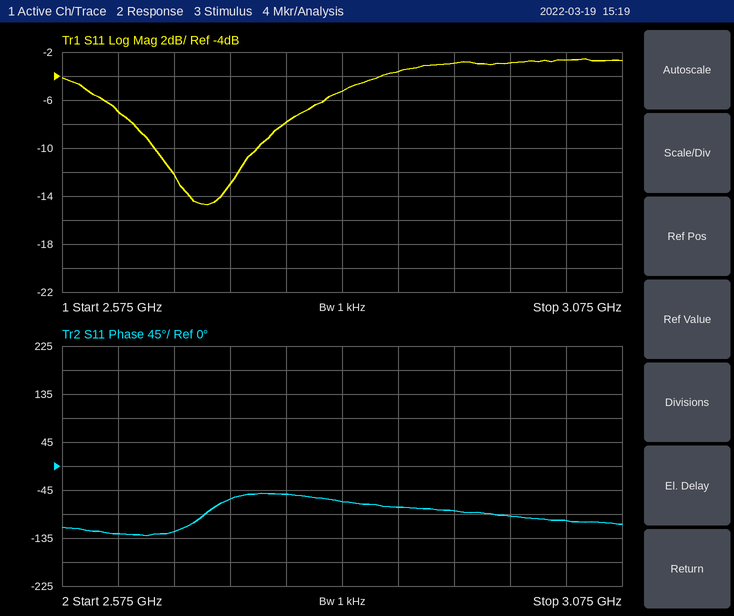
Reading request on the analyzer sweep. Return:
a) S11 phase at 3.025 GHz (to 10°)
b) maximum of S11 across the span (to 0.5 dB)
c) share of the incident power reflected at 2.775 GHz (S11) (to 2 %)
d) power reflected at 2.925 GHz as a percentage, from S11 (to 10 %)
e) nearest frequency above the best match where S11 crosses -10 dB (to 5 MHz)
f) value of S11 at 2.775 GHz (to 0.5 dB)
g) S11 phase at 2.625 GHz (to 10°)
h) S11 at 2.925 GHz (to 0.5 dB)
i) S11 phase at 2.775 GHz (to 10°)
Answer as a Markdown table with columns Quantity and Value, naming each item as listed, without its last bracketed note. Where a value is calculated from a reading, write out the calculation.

| Quantity | Value |
|---|---|
| S11 phase at 3.025 GHz | -100° |
| maximum of S11 across the span | -2.5 dB |
| share of the incident power reflected at 2.775 GHz (S11) | 10^(-8/10) ≈ 16 % |
| power reflected at 2.925 GHz as a percentage, from S11 | 10^(-3/10) ≈ 50 % |
| nearest frequency above the best match where S11 crosses -10 dB | 2.750 GHz |
| value of S11 at 2.775 GHz | -8.0 dB |
| S11 phase at 2.625 GHz | -130° |
| S11 at 2.925 GHz | -3.0 dB |
| S11 phase at 2.775 GHz | -50° |
